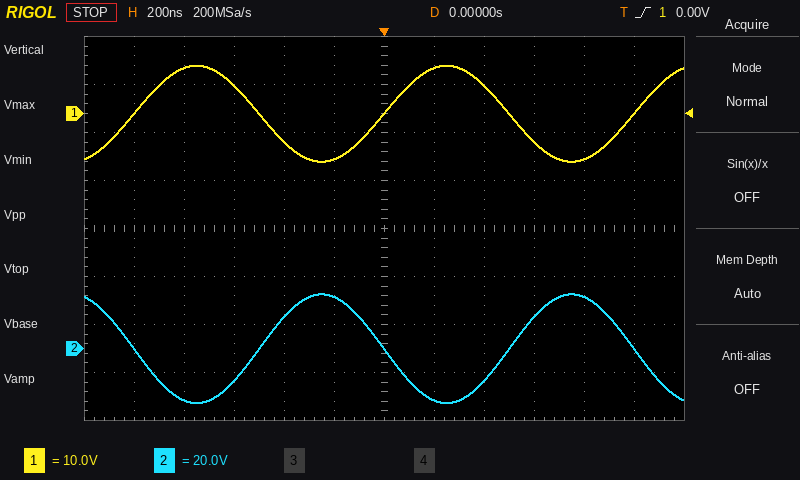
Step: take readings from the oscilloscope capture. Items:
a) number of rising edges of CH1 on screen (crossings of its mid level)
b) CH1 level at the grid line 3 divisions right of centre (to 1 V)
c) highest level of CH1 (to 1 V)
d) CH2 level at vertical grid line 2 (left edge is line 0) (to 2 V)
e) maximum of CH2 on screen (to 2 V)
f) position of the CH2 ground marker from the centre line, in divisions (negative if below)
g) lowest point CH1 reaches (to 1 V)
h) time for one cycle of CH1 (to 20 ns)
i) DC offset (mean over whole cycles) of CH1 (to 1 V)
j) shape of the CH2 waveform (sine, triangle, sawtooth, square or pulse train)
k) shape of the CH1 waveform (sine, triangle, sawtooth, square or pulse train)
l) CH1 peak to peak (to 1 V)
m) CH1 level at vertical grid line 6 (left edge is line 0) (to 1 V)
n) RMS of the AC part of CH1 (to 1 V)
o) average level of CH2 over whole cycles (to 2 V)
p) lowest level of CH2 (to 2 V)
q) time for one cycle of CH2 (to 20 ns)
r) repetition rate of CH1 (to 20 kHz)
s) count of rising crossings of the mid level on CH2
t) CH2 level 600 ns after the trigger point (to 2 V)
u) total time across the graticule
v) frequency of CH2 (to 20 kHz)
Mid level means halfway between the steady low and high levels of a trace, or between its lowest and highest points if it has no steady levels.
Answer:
3
-6 V
10 V
-22 V
22 V
-2.5 div
-10 V
1.00 µs
0 V
sine
sine
20 V
0 V
7 V
0 V
-22 V
1.00 µs
1.00 MHz
2
14 V
2.4 µs
1.00 MHz
